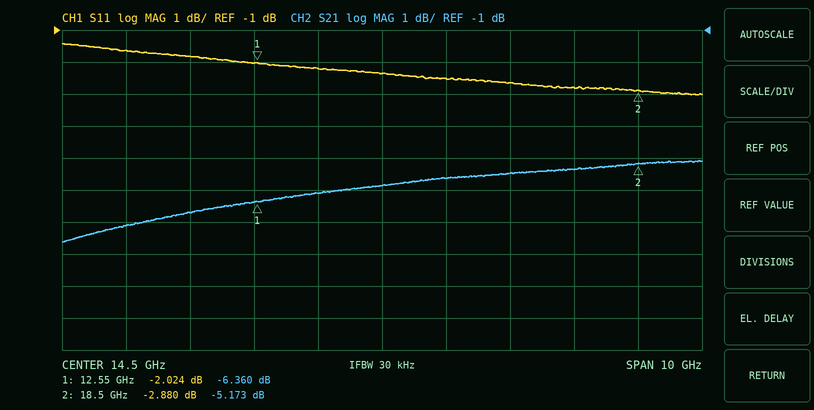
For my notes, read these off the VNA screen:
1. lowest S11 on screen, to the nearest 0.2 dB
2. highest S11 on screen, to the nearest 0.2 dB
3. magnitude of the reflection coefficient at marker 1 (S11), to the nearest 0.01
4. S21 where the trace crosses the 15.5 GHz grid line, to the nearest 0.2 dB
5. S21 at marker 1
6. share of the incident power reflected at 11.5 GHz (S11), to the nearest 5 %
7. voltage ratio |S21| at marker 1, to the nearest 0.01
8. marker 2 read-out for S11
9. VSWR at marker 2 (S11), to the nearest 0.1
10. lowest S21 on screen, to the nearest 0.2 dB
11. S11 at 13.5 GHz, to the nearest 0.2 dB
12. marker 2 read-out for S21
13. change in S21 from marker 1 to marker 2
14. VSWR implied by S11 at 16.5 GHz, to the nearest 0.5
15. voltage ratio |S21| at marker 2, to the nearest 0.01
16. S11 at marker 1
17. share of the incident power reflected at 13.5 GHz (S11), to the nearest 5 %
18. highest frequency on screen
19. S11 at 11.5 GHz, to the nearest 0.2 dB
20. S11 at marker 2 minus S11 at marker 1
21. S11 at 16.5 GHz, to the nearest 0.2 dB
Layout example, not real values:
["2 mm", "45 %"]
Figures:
["-3.0 dB", "-1.4 dB", "0.79", "-5.6 dB", "-6.360 dB", "65 %", "0.48", "-2.880 dB", "6.1", "-7.6 dB", "-2.2 dB", "-5.173 dB", "1.187 dB", "6.5", "0.55", "-2.024 dB", "60 %", "19.5 GHz", "-1.8 dB", "-0.856 dB", "-2.6 dB"]
